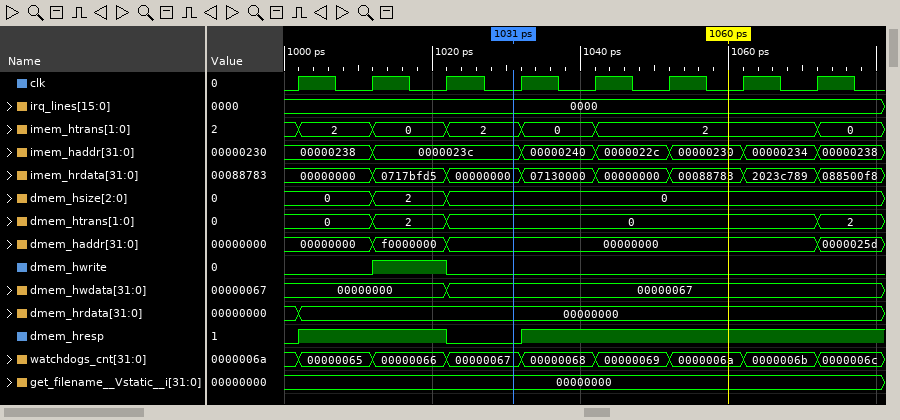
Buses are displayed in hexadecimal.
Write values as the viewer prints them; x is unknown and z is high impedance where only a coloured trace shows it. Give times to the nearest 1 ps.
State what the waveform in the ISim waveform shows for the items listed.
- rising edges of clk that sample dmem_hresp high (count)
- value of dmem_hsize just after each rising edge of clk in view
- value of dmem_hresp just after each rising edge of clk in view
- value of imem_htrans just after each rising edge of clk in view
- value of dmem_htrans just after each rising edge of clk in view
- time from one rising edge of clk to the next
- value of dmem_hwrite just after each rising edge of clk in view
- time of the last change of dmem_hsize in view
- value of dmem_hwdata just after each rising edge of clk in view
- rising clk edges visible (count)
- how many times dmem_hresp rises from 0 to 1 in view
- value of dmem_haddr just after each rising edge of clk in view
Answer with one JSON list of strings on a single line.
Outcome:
["6", "0, 2, 0, 0, 0, 0, 0, 0", "1 1 0 1 1 1 1 1", "2, 0, 2, 0, 2, 2, 2, 0", "0, 2, 0, 0, 0, 0, 0, 2", "10 ps", "0 1 0 0 0 0 0 0", "1022 ps", "00000000, 00000000, 00000067, 00000067, 00000067, 00000067, 00000067, 00000067", "8", "2", "00000000, f0000000, 00000000, 00000000, 00000000, 00000000, 00000000, 0000025d"]
